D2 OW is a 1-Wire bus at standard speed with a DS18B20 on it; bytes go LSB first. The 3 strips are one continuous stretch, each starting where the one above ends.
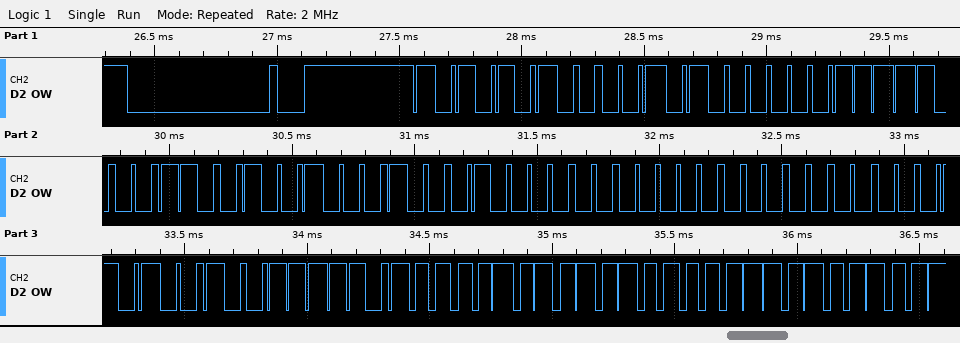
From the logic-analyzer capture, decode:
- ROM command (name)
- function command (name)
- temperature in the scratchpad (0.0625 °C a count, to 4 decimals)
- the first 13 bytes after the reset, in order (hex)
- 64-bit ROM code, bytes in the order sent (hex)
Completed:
Match ROM
Read Scratchpad
85.0000 °C
55 28 F0 31 89 08 00 00 4A BE 50 05 4B
28 F0 31 89 08 00 00 4A
